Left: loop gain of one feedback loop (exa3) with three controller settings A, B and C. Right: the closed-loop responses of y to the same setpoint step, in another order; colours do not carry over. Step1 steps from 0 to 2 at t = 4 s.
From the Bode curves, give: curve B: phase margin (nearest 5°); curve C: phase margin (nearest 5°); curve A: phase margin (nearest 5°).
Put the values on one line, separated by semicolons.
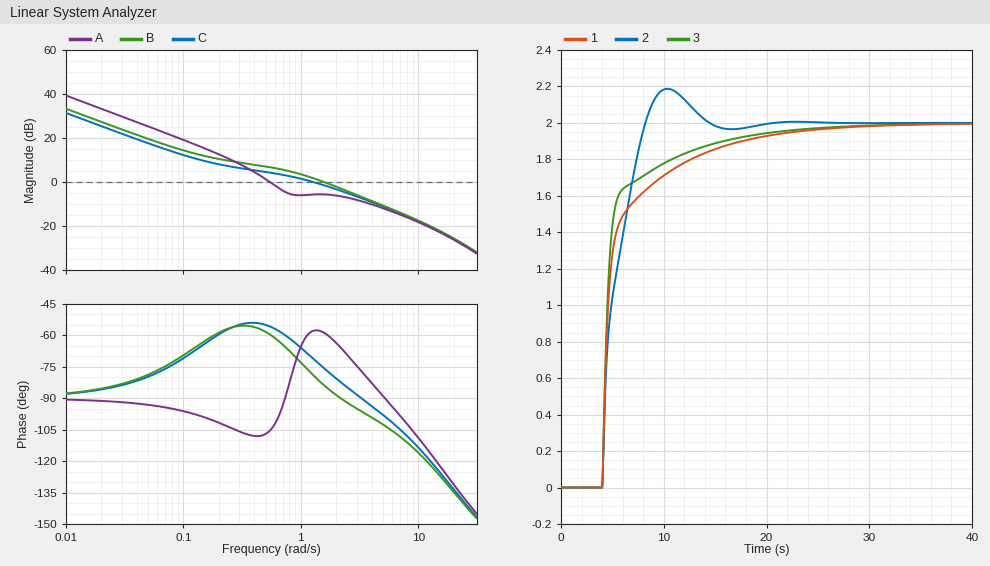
95°; 110°; 75°
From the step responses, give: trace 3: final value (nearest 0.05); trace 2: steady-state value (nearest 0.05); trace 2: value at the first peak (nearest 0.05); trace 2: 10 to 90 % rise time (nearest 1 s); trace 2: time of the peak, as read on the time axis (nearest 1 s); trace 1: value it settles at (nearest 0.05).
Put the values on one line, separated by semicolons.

2.00; 2.00; 2.20; 3 s; 10 s; 2.00
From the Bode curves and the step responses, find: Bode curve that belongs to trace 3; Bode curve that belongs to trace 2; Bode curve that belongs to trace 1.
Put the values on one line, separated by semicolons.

B; A; C
